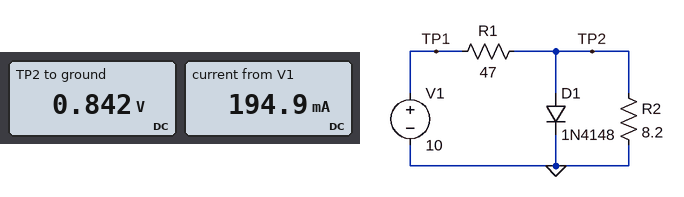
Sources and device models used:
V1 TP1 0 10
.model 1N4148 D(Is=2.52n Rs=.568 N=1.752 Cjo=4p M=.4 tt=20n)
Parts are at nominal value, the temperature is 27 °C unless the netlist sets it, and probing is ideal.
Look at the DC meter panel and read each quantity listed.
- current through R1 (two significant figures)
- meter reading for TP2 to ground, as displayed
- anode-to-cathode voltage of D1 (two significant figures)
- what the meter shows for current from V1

190 mA
0.842 V
840 mV
194.9 mA
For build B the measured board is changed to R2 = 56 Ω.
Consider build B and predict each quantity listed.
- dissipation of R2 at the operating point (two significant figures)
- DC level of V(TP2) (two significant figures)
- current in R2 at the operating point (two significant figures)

15 mW
920 mV
16 mA
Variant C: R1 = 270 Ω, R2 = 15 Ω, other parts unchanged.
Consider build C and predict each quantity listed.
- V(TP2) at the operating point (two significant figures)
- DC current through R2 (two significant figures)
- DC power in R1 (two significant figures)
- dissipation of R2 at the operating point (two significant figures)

520 mV
35 mA
330 mW
18 mW
